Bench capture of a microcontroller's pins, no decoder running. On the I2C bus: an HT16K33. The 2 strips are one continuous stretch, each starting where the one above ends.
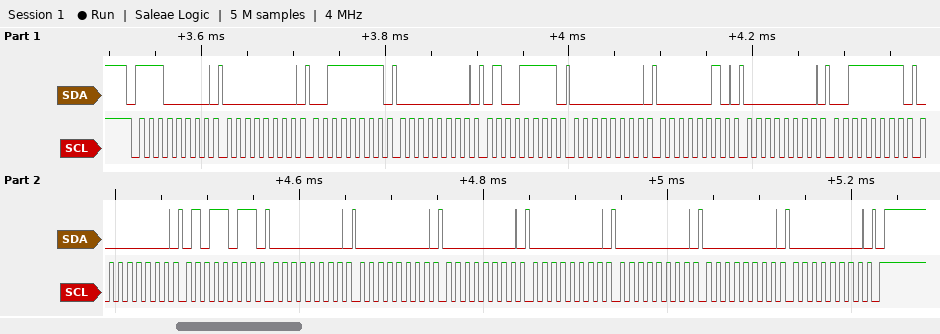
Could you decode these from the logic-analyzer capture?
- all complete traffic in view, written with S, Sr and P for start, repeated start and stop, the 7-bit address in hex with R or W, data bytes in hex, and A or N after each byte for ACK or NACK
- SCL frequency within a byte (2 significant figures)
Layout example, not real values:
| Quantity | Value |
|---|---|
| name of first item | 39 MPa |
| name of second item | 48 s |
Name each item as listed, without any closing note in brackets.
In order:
| Quantity | Value |
|---|---|
| all complete traffic in view, written with S, Sr and P for start, repeated start and stop, the 7-bit address in hex with R or W, data bytes in hex, and A or N after each byte for ACK or NACK | S 70W A 00 A 3F A 00 A 4F A 00 A 02 A 00 A 3F A 00 A 5B A 00 A 00 A 00 A 00 A 00 A 00 A 00 A P |
| SCL frequency within a byte | 100 kHz |
